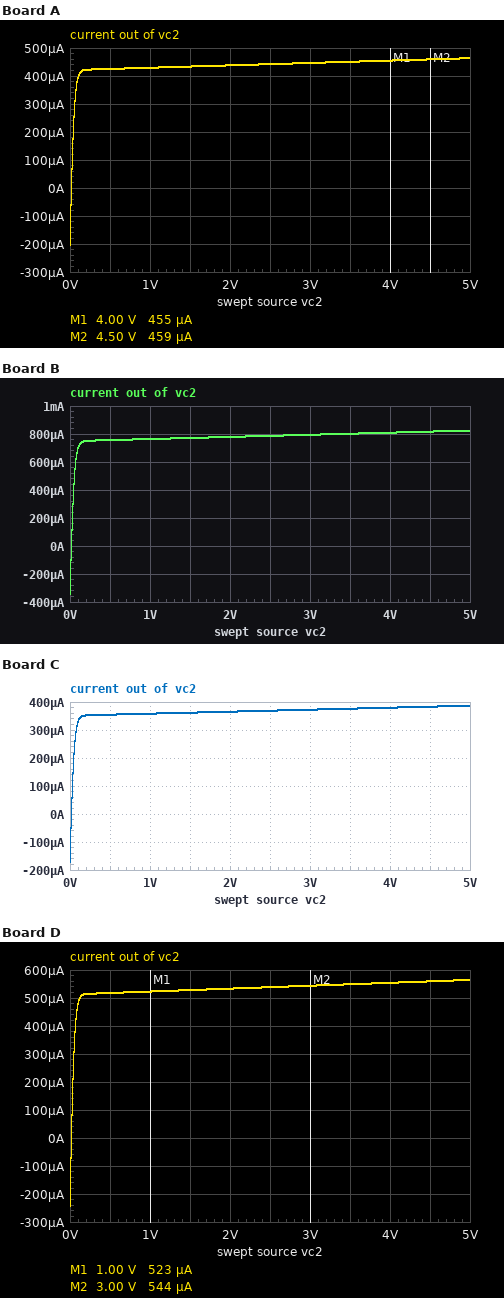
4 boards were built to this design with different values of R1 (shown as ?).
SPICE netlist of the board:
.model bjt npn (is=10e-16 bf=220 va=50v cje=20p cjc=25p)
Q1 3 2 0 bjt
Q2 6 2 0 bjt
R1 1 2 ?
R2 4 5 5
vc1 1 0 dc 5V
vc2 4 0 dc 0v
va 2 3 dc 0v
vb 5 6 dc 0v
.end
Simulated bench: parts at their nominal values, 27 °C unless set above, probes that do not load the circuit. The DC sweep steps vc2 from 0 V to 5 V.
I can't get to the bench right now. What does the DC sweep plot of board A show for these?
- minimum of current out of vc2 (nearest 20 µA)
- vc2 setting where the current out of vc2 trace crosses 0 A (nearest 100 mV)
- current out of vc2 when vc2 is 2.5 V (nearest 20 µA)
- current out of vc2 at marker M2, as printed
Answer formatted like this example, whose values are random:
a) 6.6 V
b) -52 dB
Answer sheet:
a) -200 µA
b) 0 V
c) 440 µA
d) 459 µA
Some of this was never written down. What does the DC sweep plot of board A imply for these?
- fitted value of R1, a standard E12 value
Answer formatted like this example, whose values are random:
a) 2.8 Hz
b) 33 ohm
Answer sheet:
a) 10 kΩ
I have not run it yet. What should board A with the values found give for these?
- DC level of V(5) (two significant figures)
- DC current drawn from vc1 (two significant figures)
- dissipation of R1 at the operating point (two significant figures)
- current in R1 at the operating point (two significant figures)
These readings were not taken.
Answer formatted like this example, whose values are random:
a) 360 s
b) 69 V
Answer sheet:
a) 1.0 mV
b) 430 µA
c) 1.9 mW
d) 430 µA
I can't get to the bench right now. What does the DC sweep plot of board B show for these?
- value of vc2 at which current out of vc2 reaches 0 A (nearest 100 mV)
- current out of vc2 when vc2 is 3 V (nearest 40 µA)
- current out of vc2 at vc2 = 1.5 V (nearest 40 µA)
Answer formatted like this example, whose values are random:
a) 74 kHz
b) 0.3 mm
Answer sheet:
a) 0 V
b) 800 µA
c) 760 µA
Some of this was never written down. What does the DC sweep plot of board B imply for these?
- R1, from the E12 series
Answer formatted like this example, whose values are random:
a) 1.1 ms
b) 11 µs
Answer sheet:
a) 5.6 kΩ
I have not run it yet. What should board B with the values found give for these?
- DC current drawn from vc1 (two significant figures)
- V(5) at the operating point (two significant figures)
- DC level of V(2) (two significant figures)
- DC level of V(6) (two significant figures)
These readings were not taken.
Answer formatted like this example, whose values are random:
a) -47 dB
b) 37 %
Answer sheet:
a) 770 µA
b) 1.7 mV
c) 690 mV
d) 1.7 mV
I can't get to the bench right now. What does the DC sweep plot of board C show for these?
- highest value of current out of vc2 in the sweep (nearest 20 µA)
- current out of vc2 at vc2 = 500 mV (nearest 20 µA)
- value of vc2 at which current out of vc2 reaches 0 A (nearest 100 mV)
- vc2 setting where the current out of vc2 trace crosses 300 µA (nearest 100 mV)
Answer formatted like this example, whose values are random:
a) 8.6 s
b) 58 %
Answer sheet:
a) 380 µA
b) 360 µA
c) 0 V
d) 100 mV
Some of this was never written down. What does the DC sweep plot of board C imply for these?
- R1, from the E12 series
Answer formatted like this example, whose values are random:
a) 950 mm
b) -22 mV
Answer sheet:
a) 12 kΩ
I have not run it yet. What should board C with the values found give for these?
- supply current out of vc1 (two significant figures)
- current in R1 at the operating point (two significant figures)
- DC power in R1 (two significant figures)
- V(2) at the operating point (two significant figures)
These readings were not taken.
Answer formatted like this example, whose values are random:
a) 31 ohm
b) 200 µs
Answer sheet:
a) 360 µA
b) 360 µA
c) 1.6 mW
d) 670 mV
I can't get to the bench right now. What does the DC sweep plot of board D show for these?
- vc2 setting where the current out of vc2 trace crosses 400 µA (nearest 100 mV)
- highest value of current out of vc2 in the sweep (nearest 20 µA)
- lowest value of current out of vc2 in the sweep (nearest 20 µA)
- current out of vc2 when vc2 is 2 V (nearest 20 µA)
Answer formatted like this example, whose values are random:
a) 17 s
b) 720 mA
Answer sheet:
a) 100 mV
b) 560 µA
c) -240 µA
d) 540 µA
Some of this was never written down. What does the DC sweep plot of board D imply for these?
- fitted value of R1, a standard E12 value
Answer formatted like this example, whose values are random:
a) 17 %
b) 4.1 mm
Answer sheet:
a) 8.2 kΩ
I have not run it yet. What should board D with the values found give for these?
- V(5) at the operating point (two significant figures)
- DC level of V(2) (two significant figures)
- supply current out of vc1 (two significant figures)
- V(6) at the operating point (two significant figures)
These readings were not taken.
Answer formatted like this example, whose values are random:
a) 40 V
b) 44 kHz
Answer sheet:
a) 1.2 mV
b) 680 mV
c) 530 µA
d) 1.2 mV
